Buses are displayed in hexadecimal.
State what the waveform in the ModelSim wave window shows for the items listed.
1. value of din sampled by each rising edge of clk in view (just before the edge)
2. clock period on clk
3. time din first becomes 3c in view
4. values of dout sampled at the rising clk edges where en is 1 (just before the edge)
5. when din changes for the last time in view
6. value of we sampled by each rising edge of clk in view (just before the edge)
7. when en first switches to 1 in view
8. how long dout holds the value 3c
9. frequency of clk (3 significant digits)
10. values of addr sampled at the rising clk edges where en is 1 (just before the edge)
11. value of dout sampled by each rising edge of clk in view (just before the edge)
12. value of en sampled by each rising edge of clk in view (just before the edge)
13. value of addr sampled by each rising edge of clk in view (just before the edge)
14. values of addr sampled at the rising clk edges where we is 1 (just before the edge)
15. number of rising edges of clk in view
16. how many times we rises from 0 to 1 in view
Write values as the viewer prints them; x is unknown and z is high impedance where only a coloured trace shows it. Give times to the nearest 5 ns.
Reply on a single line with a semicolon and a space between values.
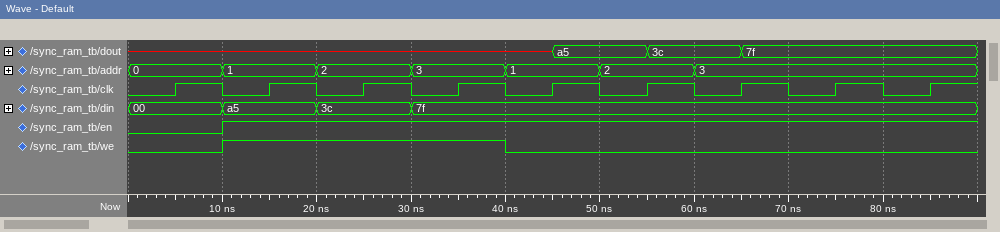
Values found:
00, a5, 3c, 7f, 7f, 7f, 7f, 7f, 7f; 10 ns; 20 ns; x, x, x, x, a5, 3c, 7f, 7f; 30 ns; 0 1 1 1 0 0 0 0 0; 10 ns; 10 ns; 100 MHz; 1, 2, 3, 1, 2, 3, 3, 3; x, x, x, x, x, a5, 3c, 7f, 7f; 0 1 1 1 1 1 1 1 1; 0, 1, 2, 3, 1, 2, 3, 3, 3; 1, 2, 3; 9; 1
